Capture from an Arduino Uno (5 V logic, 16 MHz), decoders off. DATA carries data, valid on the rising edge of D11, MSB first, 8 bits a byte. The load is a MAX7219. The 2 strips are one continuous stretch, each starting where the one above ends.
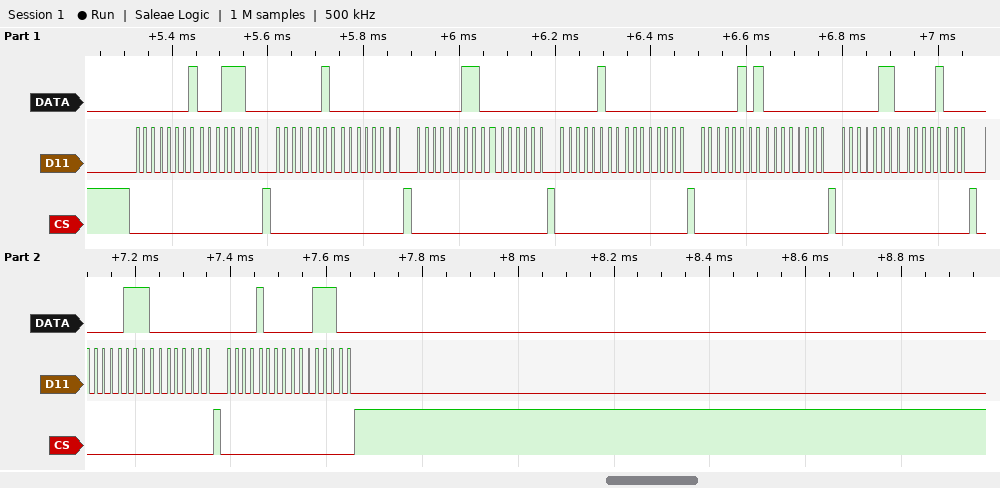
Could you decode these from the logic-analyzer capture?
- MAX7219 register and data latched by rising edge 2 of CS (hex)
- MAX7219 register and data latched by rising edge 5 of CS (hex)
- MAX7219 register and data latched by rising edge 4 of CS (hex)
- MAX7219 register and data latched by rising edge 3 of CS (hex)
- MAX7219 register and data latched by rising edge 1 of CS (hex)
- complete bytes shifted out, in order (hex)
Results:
register 0x2, data 0x00
register 0x5, data 0x00
register 0x4, data 0x00
register 0x3, data 0x00
register 0x1, data 0x1C
0x01 0x1C 0x02 0x00 0x03 0x00 0x04 0x00 0x05 0x00 0x06 0x08 0x07 0x00 0x08 0x1C
